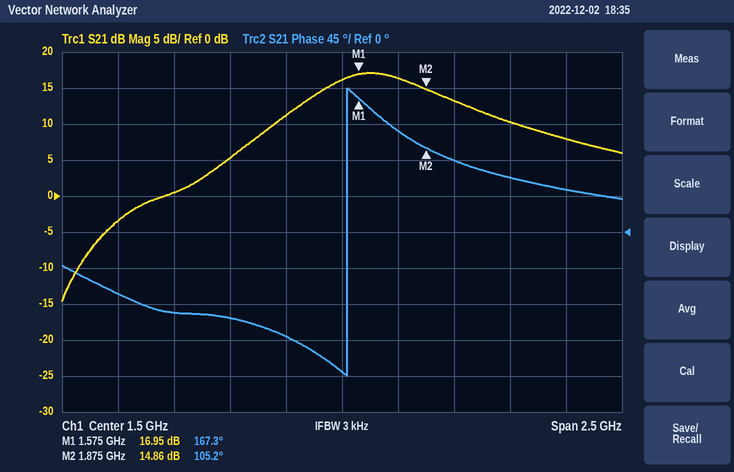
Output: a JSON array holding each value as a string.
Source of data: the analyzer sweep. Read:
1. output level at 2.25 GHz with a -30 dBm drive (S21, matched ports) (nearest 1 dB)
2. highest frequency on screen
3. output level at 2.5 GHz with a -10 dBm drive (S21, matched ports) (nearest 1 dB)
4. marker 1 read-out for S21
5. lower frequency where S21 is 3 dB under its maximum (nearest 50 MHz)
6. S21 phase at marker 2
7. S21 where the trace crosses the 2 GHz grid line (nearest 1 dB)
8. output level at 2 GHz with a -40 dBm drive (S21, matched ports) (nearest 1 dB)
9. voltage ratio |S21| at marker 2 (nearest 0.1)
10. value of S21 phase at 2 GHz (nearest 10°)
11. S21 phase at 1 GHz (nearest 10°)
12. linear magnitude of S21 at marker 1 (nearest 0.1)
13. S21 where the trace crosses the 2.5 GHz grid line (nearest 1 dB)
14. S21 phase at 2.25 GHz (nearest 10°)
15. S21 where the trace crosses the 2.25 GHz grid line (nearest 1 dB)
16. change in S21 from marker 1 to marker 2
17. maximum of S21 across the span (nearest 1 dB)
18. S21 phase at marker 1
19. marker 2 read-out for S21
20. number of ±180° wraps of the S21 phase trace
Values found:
["-20 dBm", "2.75 GHz", "-2 dBm", "16.95 dB", "1.40 GHz", "105.2°", "13 dB", "-27 dBm", "5.5", "90°", "-110°", "7.0", "8 dB", "70°", "10 dB", "-2.09 dB", "17 dB", "167.3°", "14.86 dB", "1"]
